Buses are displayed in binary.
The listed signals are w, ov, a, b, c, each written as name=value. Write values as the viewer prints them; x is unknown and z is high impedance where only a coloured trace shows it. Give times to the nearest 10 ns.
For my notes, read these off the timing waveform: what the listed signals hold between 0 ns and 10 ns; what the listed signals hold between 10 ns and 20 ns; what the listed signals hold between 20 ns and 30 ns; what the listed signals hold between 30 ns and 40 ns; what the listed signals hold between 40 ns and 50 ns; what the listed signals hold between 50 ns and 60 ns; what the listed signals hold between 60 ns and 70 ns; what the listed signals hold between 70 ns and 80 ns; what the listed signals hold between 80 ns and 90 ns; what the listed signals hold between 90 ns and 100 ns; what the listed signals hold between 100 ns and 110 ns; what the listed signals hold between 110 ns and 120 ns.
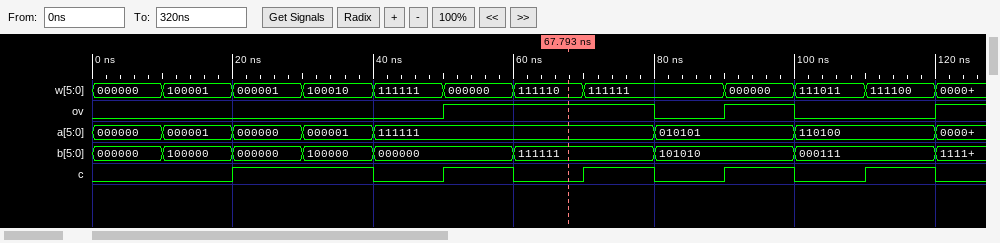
w=000000, ov=0, a=000000, b=000000, c=0
w=100001, ov=0, a=000001, b=100000, c=0
w=000001, ov=0, a=000000, b=000000, c=1
w=100010, ov=0, a=000001, b=100000, c=1
w=111111, ov=0, a=111111, b=000000, c=0
w=000000, ov=1, a=111111, b=000000, c=1
w=111110, ov=1, a=111111, b=111111, c=0
w=111111, ov=1, a=111111, b=111111, c=1
w=111111, ov=0, a=010101, b=101010, c=0
w=000000, ov=1, a=010101, b=101010, c=1
w=111011, ov=0, a=110100, b=000111, c=0
w=111100, ov=0, a=110100, b=000111, c=1
